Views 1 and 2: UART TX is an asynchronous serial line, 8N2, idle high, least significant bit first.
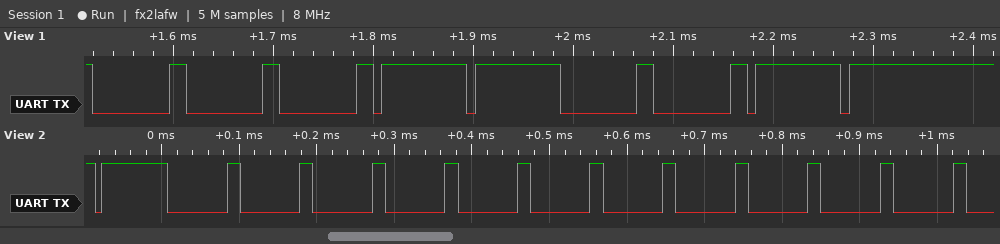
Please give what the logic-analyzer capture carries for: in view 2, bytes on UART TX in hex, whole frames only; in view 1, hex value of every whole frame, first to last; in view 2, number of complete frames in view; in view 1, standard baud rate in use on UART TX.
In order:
FF 00 00 00 00 00 00 00 00 00 00 00
0x00 0x00 0x00 0xFF 0xFF 0x00 0x00 0xFF 0xFF
12
115200 baud
